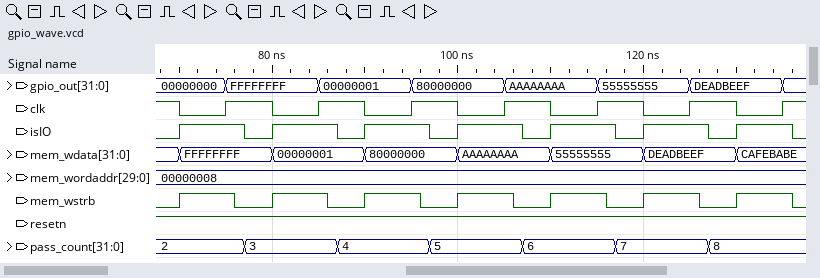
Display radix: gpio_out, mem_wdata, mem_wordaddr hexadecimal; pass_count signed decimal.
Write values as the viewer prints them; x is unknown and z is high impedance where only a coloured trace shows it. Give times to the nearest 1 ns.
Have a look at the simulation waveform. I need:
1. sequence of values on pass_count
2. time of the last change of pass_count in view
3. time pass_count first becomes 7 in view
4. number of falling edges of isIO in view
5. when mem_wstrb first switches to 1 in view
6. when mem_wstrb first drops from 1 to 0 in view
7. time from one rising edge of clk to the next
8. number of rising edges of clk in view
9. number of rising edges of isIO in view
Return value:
2, 3, 4, 5, 6, 7, 8
127 ns
117 ns
7
70 ns
76 ns
10 ns
7
7
